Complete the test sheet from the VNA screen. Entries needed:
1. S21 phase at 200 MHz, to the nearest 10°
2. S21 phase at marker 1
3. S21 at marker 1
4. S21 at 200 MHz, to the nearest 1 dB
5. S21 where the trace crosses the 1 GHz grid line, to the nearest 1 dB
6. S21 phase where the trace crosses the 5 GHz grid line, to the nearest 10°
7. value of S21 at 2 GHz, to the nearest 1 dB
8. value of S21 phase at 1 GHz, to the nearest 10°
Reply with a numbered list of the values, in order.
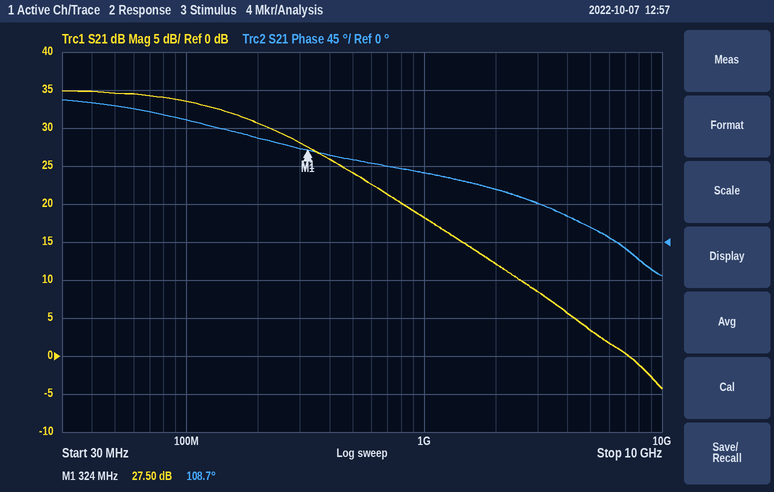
1. 120°
2. 108.7°
3. 27.50 dB
4. 31 dB
5. 18 dB
6. 20°
7. 12 dB
8. 80°
